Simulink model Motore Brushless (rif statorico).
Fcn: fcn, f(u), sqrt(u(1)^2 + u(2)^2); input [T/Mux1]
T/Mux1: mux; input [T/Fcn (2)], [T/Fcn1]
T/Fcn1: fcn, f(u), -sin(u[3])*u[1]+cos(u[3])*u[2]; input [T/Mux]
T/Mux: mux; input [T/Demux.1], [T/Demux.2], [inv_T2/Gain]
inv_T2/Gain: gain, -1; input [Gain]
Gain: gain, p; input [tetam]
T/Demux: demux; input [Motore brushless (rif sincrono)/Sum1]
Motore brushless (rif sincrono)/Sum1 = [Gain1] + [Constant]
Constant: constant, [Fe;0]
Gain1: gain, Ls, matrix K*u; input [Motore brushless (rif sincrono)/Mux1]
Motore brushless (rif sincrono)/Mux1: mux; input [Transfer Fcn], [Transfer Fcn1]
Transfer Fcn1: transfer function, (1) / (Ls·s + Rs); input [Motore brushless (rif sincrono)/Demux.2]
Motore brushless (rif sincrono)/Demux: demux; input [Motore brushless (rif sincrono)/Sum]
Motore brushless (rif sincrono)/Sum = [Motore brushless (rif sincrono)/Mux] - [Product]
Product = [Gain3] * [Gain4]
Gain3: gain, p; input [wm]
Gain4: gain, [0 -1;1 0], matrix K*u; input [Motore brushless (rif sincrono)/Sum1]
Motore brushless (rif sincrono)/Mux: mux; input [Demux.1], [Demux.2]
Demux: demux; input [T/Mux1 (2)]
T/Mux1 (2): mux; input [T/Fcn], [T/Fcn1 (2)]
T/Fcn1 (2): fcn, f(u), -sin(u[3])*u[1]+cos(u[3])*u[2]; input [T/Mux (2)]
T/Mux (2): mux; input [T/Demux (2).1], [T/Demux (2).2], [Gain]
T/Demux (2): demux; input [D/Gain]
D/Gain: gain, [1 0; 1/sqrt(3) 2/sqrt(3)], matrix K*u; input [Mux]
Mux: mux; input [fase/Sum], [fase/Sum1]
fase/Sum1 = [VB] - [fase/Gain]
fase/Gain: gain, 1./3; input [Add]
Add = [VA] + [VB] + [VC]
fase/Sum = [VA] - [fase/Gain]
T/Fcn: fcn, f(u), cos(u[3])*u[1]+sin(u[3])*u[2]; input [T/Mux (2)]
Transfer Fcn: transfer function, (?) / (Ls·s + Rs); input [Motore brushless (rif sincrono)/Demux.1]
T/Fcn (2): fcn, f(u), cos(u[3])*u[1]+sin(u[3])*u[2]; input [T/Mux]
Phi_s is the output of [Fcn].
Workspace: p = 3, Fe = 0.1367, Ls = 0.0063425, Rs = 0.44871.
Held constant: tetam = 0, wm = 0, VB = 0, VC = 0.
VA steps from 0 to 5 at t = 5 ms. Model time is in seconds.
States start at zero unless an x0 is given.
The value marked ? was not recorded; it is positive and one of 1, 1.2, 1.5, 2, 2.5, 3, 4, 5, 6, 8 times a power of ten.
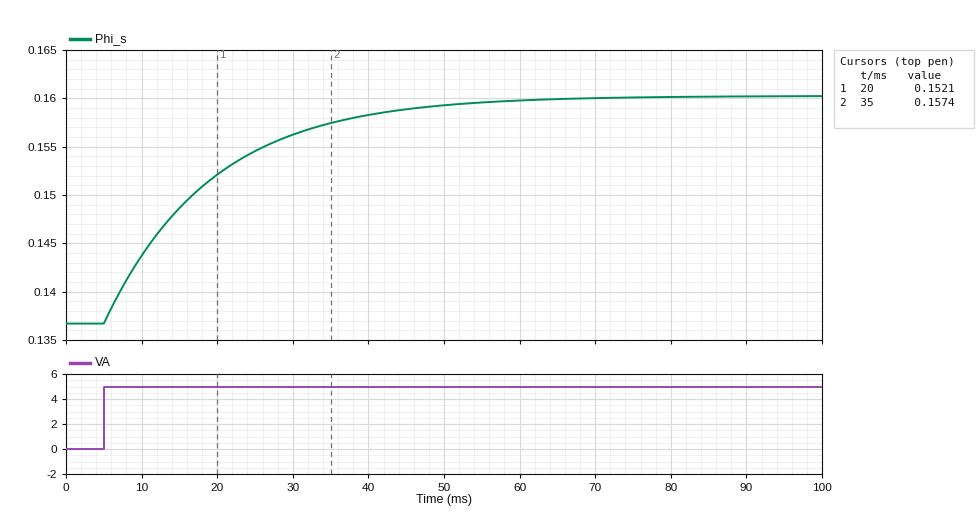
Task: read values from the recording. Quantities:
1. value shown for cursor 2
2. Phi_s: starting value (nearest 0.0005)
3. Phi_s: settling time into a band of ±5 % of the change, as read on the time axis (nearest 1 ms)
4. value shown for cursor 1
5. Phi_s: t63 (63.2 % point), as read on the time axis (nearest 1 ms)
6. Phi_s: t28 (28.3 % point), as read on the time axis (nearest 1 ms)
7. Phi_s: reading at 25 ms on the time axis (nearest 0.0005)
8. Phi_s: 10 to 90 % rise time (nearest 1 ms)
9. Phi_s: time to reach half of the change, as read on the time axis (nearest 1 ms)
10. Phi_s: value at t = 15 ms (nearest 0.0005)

0.1574
0.1365
47 ms
0.1521
19 ms
10 ms
0.1545
31 ms
15 ms
0.1485
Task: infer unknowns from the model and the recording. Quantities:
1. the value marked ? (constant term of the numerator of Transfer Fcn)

0.5
